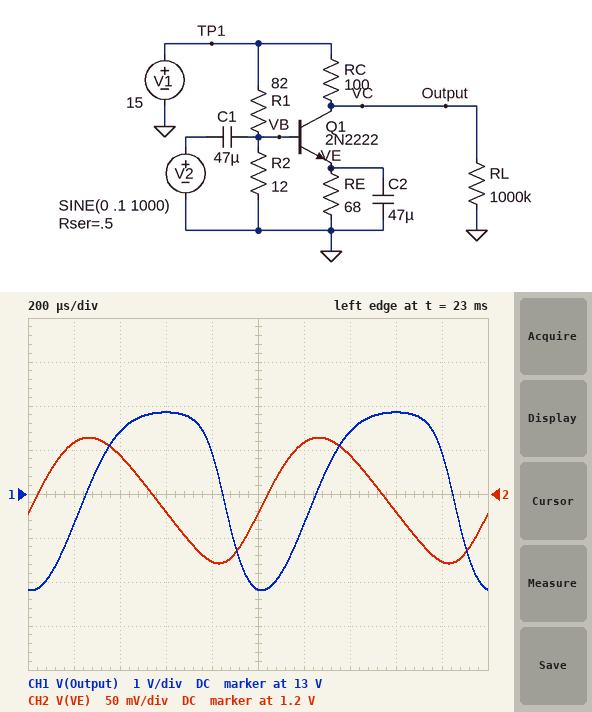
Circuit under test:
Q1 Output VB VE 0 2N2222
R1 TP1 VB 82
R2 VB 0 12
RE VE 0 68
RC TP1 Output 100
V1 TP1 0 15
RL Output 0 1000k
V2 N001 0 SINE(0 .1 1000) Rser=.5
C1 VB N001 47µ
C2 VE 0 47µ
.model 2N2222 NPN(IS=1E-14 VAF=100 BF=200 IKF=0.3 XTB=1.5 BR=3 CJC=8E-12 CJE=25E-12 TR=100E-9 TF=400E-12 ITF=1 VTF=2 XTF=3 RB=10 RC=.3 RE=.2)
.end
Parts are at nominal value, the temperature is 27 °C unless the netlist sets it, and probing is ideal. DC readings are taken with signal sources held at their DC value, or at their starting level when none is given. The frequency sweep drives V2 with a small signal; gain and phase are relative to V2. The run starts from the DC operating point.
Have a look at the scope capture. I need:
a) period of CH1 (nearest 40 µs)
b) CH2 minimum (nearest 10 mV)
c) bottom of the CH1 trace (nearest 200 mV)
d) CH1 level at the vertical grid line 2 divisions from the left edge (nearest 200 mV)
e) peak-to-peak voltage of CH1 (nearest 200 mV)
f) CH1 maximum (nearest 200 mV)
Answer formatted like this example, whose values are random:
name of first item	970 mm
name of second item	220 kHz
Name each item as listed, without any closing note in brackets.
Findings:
period of CH1	1.00 ms
CH2 minimum	1.12 V
bottom of the CH1 trace	10.8 V
CH1 level at the vertical grid line 2 divisions from the left edge	14.4 V
peak-to-peak voltage of CH1	4.0 V
CH1 maximum	14.8 V
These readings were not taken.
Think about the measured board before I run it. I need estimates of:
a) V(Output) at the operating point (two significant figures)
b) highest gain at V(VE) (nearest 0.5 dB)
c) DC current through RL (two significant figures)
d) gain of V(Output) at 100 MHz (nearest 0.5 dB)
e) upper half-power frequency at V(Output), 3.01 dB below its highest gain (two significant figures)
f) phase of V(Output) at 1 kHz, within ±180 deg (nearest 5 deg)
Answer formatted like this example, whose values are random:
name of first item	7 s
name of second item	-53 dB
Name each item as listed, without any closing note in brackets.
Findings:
V(Output) at the operating point	13 V
highest gain at V(VE)	-2.0 dB
DC current through RL	13 µA
gain of V(Output) at 100 MHz	24.5 dB
upper half-power frequency at V(Output), 3.01 dB below its highest gain	34 MHz
phase of V(Output) at 1 kHz, within ±180 deg	-105 deg
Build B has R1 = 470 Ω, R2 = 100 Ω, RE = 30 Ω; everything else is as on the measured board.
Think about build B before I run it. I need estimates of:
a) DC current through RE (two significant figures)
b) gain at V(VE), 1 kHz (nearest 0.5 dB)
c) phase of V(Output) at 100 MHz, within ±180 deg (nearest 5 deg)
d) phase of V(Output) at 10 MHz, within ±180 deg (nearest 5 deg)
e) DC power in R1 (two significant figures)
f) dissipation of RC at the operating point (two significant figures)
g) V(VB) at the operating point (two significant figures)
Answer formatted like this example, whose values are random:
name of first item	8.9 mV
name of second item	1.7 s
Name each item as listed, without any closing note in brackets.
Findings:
DC current through RE	61 mA
gain at V(VE), 1 kHz	-0.5 dB
phase of V(Output) at 100 MHz, within ±180 deg	90 deg
phase of V(Output) at 10 MHz, within ±180 deg	145 deg
DC power in R1	330 mW
dissipation of RC at the operating point	370 mW
V(VB) at the operating point	2.6 V
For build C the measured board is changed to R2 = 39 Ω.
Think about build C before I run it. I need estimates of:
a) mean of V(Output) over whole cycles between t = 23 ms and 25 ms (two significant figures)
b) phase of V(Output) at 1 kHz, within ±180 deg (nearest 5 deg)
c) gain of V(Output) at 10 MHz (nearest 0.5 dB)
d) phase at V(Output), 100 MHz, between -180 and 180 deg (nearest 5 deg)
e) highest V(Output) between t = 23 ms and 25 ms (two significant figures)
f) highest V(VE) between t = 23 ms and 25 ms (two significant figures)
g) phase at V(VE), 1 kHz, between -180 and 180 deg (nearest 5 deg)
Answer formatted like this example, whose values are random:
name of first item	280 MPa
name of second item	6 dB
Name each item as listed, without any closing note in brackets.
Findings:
mean of V(Output) over whole cycles between t = 23 ms and 25 ms	9.1 V
phase of V(Output) at 1 kHz, within ±180 deg	-100 deg
gain of V(Output) at 10 MHz	40.0 dB
phase at V(Output), 100 MHz, between -180 and 180 deg	90 deg
highest V(Output) between t = 23 ms and 25 ms	12 V
highest V(VE) between t = 23 ms and 25 ms	4.1 V
phase at V(VE), 1 kHz, between -180 and 180 deg	-5 deg
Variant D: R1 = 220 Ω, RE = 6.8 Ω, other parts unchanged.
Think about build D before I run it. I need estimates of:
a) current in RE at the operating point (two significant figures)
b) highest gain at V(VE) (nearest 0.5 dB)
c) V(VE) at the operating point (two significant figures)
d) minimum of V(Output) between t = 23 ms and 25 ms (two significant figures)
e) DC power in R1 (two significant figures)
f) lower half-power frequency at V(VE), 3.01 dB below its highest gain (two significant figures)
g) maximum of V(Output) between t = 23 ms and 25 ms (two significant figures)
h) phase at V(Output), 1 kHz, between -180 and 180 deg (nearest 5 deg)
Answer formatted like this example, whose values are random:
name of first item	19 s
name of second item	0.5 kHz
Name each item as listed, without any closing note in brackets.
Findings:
current in RE at the operating point	9.3 mA
highest gain at V(VE)	-5.0 dB
V(VE) at the operating point	63 mV
minimum of V(Output) between t = 23 ms and 25 ms	12 V
DC power in R1	920 mW
lower half-power frequency at V(VE), 3.01 dB below its highest gain	220 Hz
maximum of V(Output) between t = 23 ms and 25 ms	15 V
phase at V(Output), 1 kHz, between -180 and 180 deg	-135 deg
